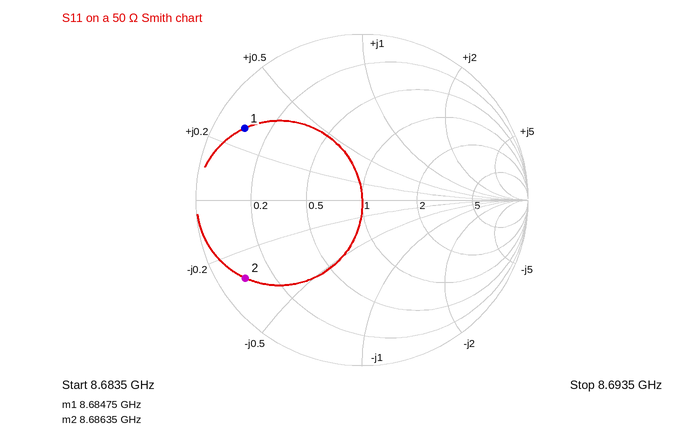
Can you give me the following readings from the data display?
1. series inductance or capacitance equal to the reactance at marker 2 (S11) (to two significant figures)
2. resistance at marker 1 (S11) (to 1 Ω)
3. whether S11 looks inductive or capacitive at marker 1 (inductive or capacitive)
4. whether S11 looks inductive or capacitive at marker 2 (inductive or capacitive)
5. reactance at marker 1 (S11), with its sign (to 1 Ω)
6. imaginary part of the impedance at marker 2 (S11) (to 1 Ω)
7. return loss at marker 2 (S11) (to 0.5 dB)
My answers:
1.2 pF
5 Ω
inductive
capacitive
+14 Ω
-15 Ω
1.5 dB
